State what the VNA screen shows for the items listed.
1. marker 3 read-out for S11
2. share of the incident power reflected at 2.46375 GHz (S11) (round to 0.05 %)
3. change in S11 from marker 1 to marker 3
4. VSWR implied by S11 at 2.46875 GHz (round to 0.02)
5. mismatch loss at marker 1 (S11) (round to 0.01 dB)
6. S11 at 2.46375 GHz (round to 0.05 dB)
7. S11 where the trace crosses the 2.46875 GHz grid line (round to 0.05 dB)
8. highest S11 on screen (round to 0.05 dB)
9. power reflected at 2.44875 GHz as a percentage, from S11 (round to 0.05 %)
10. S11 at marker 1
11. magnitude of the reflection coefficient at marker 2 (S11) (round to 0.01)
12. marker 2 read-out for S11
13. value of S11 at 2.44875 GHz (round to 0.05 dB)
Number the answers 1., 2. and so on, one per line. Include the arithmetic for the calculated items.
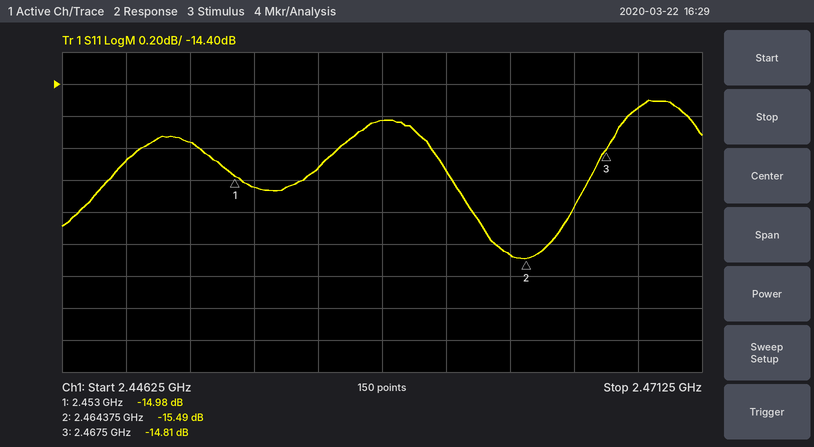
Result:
1. -14.81 dB
2. 10^(-15.45/10) ≈ 2.85 %
3. -14.81 − (-14.98) = 0.17 dB
4. |Γ| = 10^(-14.55/20) = 0.1873; VSWR = (1 + 0.1873)/(1 − 0.1873) ≈ 1.46
5. −10 log10(1 − 10^(-14.98/10)) ≈ 0.14 dB
6. -15.45 dB
7. -14.55 dB
8. -14.50 dB
9. 10^(-14.9/10) ≈ 3.24 %, so 3.25 % to the nearest 0.05 %
10. -14.98 dB
11. 10^(-15.49/20) ≈ 0.17
12. -15.49 dB
13. -14.90 dB
